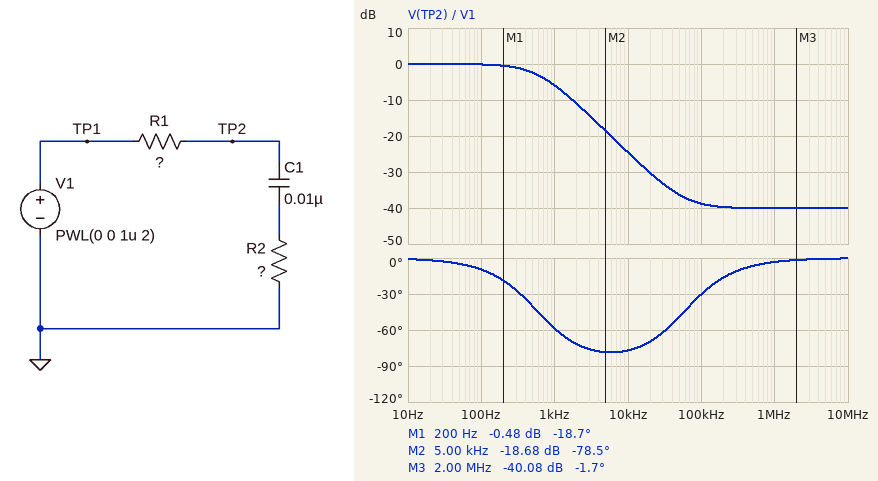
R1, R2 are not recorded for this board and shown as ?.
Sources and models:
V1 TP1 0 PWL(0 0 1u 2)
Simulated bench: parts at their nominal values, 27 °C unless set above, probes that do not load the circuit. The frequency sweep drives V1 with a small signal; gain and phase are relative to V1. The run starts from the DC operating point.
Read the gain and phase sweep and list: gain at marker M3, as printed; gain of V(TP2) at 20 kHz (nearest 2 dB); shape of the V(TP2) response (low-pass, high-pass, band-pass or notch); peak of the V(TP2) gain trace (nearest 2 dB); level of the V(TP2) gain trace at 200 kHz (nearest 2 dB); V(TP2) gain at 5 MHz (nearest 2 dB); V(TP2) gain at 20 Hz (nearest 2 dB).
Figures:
-40.08 dB
-30 dB
low-pass
0 dB
-40 dB
-40 dB
0 dB
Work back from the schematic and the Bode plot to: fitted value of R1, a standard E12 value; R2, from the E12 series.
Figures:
27 kΩ
270 Ω
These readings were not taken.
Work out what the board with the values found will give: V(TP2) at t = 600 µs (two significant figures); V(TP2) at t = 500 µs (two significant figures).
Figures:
1.8 V
1.7 V
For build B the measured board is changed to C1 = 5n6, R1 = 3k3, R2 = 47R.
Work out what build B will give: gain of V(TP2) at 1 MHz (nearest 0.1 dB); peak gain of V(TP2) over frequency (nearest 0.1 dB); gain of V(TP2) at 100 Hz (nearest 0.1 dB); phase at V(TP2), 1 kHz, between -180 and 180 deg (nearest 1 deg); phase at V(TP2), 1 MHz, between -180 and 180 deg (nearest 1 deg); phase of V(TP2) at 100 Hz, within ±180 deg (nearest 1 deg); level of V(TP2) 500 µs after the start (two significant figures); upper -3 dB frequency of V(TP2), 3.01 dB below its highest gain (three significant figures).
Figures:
-35.7 dB
0 dB
0 dB
-7 deg
-31 deg
-1 deg
2.0 V
8.49 kHz
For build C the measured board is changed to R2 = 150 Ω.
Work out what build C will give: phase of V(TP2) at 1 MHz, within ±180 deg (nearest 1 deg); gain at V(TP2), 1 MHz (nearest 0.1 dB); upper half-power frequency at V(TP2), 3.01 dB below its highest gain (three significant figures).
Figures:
-6 deg
-45.1 dB
586 Hz
